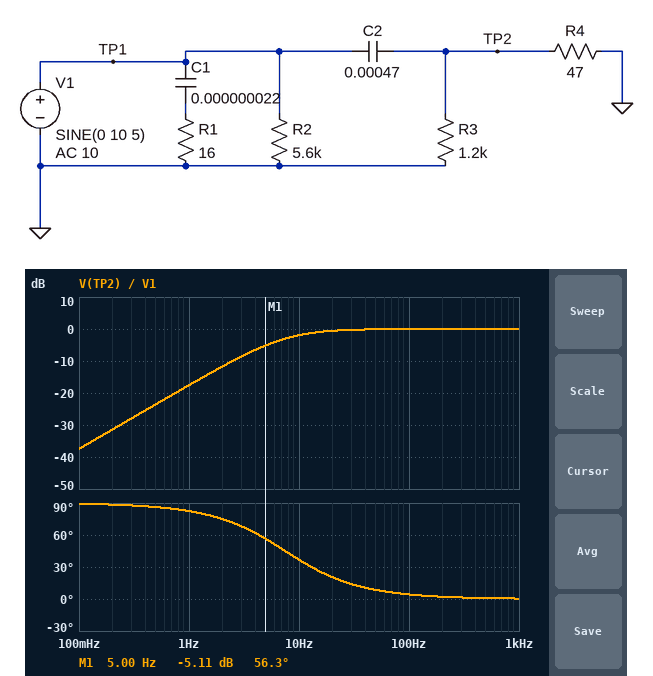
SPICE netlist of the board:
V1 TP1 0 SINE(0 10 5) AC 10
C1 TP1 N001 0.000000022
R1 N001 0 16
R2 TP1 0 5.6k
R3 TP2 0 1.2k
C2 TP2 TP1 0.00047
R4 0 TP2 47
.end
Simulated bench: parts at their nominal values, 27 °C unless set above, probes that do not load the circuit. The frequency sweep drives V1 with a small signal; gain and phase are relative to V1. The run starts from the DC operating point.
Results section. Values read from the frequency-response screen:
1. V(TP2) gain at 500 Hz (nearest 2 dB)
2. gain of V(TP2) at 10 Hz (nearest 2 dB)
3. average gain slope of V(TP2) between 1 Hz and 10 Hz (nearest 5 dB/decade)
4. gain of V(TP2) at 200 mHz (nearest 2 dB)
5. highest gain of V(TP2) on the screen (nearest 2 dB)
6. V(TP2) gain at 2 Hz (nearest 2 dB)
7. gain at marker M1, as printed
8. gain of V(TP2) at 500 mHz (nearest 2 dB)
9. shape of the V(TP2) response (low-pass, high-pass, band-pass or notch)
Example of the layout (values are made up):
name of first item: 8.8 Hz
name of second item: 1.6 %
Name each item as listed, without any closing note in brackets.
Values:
V(TP2) gain at 500 Hz: 0 dB
gain of V(TP2) at 10 Hz: -2 dB
average gain slope of V(TP2) between 1 Hz and 10 Hz: 15 dB/decade
gain of V(TP2) at 200 mHz: -32 dB
highest gain of V(TP2) on the screen: 0 dB
V(TP2) gain at 2 Hz: -12 dB
gain at marker M1, as printed: -5.11 dB
gain of V(TP2) at 500 mHz: -24 dB
shape of the V(TP2) response: high-pass
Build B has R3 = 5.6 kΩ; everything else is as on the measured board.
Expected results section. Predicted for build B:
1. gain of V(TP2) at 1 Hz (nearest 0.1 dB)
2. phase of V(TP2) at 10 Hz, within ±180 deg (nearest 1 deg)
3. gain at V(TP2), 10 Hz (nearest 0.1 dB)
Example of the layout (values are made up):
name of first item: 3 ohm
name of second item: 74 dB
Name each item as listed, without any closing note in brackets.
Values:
gain of V(TP2) at 1 Hz: -17.3 dB
phase of V(TP2) at 10 Hz, within ±180 deg: 36 deg
gain at V(TP2), 10 Hz: -1.8 dB
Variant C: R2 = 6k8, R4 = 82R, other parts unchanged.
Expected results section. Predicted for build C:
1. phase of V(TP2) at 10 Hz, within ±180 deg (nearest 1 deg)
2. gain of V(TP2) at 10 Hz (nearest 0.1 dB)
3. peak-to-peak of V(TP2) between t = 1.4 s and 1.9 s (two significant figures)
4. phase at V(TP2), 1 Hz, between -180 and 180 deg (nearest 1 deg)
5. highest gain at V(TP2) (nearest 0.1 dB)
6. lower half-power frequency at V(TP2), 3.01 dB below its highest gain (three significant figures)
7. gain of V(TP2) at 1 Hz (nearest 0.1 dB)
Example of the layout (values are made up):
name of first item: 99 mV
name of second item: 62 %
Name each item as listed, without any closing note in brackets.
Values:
phase of V(TP2) at 10 Hz, within ±180 deg: 24 deg
gain of V(TP2) at 10 Hz: -0.8 dB
peak-to-peak of V(TP2) between t = 1.4 s and 1.9 s: 15 V
phase at V(TP2), 1 Hz, between -180 and 180 deg: 77 deg
highest gain at V(TP2): 0 dB
lower half-power frequency at V(TP2), 3.01 dB below its highest gain: 4.41 Hz
gain of V(TP2) at 1 Hz: -13.1 dB
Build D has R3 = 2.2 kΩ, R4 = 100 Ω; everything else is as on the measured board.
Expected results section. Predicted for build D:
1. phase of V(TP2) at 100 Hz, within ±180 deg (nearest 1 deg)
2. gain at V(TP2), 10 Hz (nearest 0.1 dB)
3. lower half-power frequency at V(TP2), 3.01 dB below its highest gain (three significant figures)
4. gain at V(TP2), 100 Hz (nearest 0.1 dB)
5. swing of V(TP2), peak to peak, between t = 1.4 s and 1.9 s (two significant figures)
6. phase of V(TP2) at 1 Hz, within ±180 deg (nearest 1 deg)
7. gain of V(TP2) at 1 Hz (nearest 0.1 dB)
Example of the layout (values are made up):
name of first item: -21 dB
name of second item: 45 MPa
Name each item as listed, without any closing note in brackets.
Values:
phase of V(TP2) at 100 Hz, within ±180 deg: 2 deg
gain at V(TP2), 10 Hz: -0.5 dB
lower half-power frequency at V(TP2), 3.01 dB below its highest gain: 3.54 Hz
gain at V(TP2), 100 Hz: 0 dB
swing of V(TP2), peak to peak, between t = 1.4 s and 1.9 s: 16 V
phase of V(TP2) at 1 Hz, within ±180 deg: 74 deg
gain of V(TP2) at 1 Hz: -11.3 dB
